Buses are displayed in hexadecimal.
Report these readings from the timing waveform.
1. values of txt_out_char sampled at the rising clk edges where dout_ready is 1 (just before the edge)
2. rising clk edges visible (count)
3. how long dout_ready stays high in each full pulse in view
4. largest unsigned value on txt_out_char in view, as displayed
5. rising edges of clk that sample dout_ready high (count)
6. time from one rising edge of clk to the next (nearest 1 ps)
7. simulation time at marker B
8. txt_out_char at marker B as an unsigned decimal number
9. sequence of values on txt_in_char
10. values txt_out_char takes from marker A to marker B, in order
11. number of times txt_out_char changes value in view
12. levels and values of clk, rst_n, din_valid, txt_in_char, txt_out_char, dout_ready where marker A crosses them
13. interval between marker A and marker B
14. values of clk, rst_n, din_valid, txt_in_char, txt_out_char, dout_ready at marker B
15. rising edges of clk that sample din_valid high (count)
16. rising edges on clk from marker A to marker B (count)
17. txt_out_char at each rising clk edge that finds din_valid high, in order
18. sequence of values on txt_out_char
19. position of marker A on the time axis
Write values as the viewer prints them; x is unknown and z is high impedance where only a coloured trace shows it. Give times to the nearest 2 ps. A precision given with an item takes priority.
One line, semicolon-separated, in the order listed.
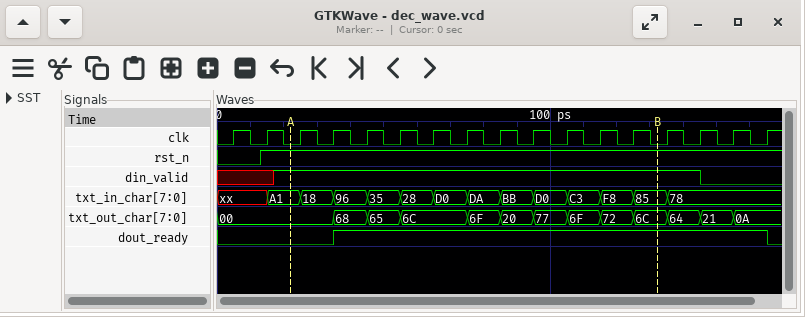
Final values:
68, 65, 6C, 6C, 6F, 20, 77, 6F, 72, 6C, 64, 21, 0A; 17; 130 ps; 77; 13; 10 ps; 132 ps; 108; xx, A1, 18, 96, 35, 28, D0, DA, BB, D0, C3, F8, 85, 78; 00, 68, 65, 6C, 6F, 20, 77, 6F, 72, 6C; 12; clk=0, rst_n=1, din_valid=1, txt_in_char=A1, txt_out_char=00, dout_ready=0; 110 ps; clk=0, rst_n=1, din_valid=1, txt_in_char=85, txt_out_char=6C, dout_ready=1; 13; 11; 00, 00, 68, 65, 6C, 6C, 6F, 20, 77, 6F, 72, 6C, 64; 00, 68, 65, 6C, 6F, 20, 77, 6F, 72, 6C, 64, 21, 0A; 22 ps
